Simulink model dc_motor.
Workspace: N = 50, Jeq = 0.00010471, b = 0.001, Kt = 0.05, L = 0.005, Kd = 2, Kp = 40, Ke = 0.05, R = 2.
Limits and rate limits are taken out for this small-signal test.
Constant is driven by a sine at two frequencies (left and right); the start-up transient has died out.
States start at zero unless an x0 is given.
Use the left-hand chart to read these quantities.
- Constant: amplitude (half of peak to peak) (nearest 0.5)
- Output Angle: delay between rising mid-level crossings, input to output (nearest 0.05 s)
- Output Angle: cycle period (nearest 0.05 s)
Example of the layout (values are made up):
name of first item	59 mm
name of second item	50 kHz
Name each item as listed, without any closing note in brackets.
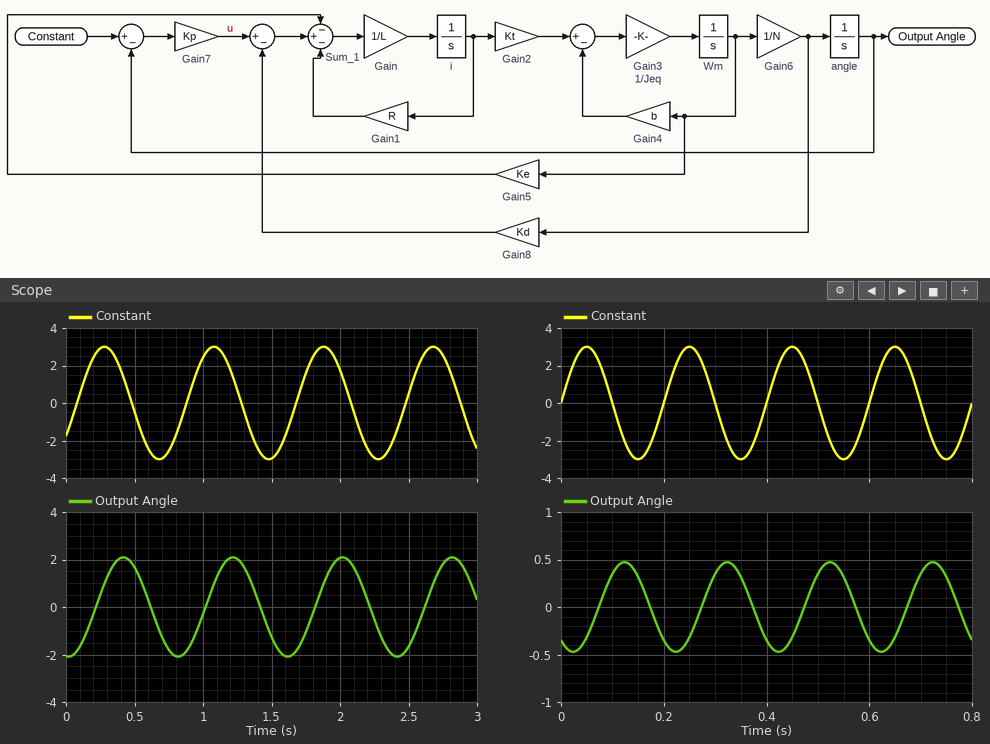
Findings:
Constant: amplitude (half of peak to peak)	3.0
Output Angle: delay between rising mid-level crossings, input to output	0.15 s
Output Angle: cycle period	0.80 s
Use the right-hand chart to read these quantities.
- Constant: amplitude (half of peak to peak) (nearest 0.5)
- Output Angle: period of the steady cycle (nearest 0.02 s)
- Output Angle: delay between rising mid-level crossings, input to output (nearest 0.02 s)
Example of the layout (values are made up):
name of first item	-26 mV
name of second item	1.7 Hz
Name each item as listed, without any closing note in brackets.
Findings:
Constant: amplitude (half of peak to peak)	3.0
Output Angle: period of the steady cycle	0.20 s
Output Angle: delay between rising mid-level crossings, input to output	0.08 s
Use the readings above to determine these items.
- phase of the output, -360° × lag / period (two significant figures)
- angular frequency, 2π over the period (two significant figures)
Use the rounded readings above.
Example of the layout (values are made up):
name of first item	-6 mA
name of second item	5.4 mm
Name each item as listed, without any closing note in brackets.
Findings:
phase of the output, -360° × lag / period	-140°
angular frequency, 2π over the period	31 rad/s
